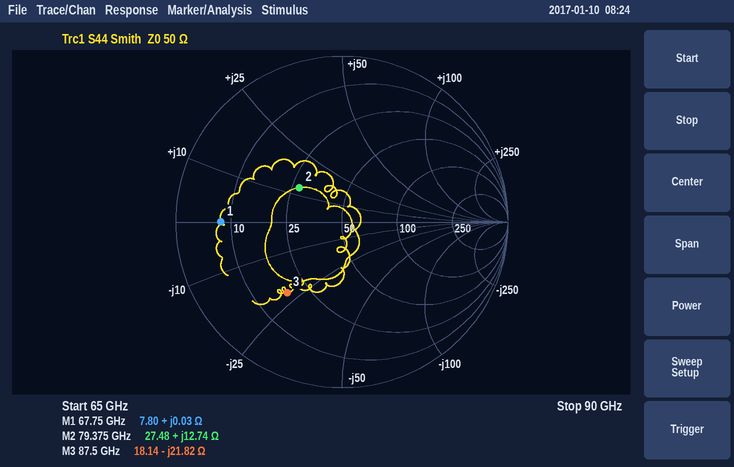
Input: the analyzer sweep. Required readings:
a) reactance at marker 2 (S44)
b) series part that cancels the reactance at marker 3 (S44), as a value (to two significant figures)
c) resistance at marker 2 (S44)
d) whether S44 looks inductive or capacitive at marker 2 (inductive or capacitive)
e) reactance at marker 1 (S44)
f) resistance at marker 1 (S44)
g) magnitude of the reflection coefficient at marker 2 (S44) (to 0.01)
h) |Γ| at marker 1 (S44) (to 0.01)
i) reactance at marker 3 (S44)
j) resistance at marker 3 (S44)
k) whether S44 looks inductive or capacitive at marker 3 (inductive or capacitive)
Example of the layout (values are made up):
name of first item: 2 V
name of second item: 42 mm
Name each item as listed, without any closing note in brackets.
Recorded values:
reactance at marker 2: +12.74 Ω
series part that cancels the reactance at marker 3 (S44), as a value: 40 pH
resistance at marker 2: 27.48 Ω
whether S44 looks inductive or capacitive at marker 2: inductive
reactance at marker 1: +0.03 Ω
resistance at marker 1: 7.80 Ω
magnitude of the reflection coefficient at marker 2 (S44): 0.33
|Γ| at marker 1 (S44): 0.73
reactance at marker 3: -21.82 Ω
resistance at marker 3: 18.14 Ω
whether S44 looks inductive or capacitive at marker 3: capacitive
